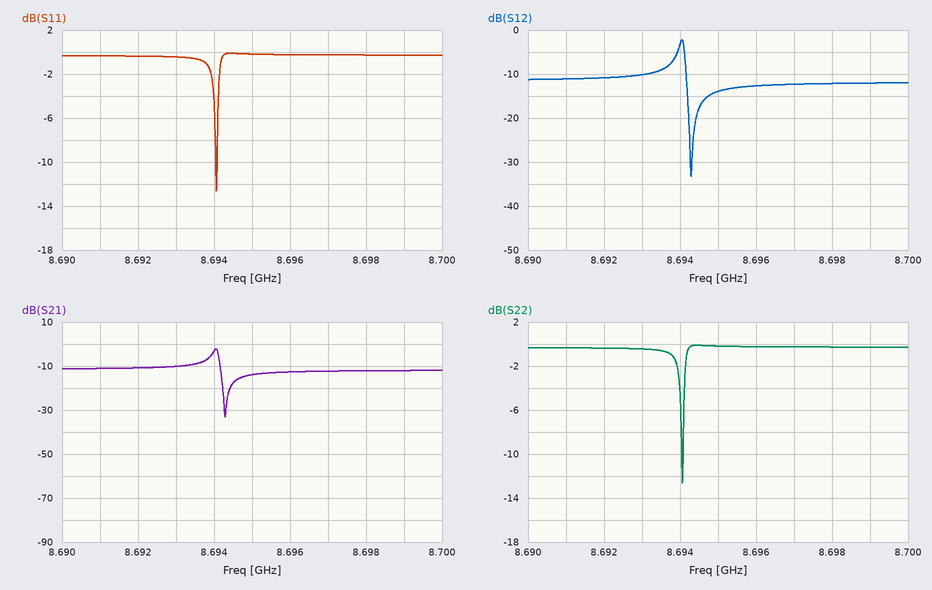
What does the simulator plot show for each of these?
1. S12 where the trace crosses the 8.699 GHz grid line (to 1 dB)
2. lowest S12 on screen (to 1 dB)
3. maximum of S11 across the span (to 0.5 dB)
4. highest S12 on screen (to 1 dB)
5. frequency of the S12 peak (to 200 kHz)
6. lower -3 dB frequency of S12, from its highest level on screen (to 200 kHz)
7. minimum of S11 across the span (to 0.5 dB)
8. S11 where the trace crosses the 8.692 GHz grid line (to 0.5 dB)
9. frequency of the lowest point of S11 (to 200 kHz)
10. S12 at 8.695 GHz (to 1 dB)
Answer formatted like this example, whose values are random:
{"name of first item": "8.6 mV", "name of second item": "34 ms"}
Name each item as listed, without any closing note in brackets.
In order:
{"S12 where the trace crosses the 8.699 GHz grid line": "-12 dB", "lowest S12 on screen": "-33 dB", "maximum of S11 across the span": "0.0 dB", "highest S12 on screen": "-2 dB", "frequency of the S12 peak": "8.6940 GHz", "lower -3 dB frequency of S12, from its highest level on screen": "8.6940 GHz", "minimum of S11 across the span": "-12.5 dB", "S11 where the trace crosses the 8.692 GHz grid line": "-0.5 dB", "frequency of the lowest point of S11": "8.6940 GHz", "S12 at 8.695 GHz": "-14 dB"}
